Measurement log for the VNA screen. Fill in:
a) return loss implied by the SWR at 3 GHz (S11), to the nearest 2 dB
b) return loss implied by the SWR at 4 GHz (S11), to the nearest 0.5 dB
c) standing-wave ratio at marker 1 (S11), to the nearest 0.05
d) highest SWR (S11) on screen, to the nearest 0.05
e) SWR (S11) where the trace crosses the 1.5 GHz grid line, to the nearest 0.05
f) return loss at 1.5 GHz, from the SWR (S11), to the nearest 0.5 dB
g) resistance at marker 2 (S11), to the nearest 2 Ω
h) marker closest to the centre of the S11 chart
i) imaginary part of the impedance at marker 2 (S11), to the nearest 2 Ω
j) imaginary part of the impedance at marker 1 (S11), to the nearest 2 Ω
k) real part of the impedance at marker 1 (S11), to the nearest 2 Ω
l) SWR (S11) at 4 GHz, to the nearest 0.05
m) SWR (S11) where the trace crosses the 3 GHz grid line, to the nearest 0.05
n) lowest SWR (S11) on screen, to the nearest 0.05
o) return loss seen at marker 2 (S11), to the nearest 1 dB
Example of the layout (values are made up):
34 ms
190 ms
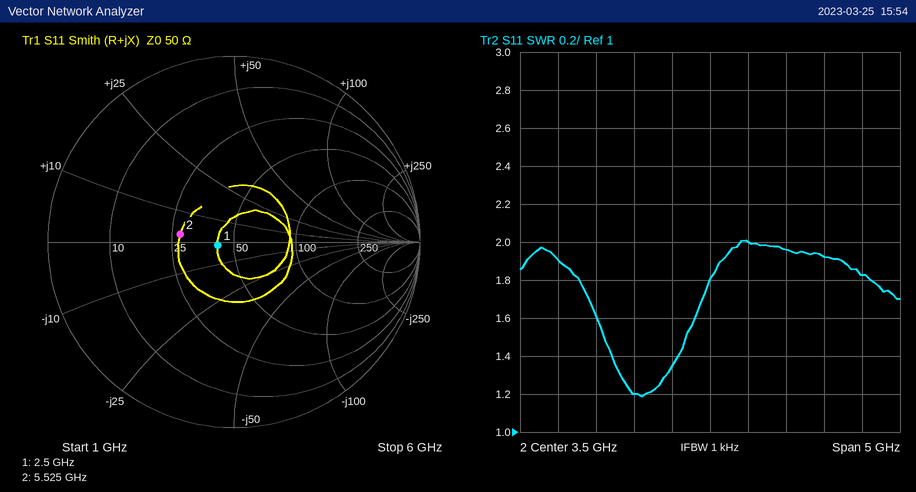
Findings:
16 dB
9.5 dB
1.20
2.00
1.90
10.0 dB
28 Ω
marker 1
+2 Ω
-2 Ω
42 Ω
2.00
1.35
1.20
11 dB
